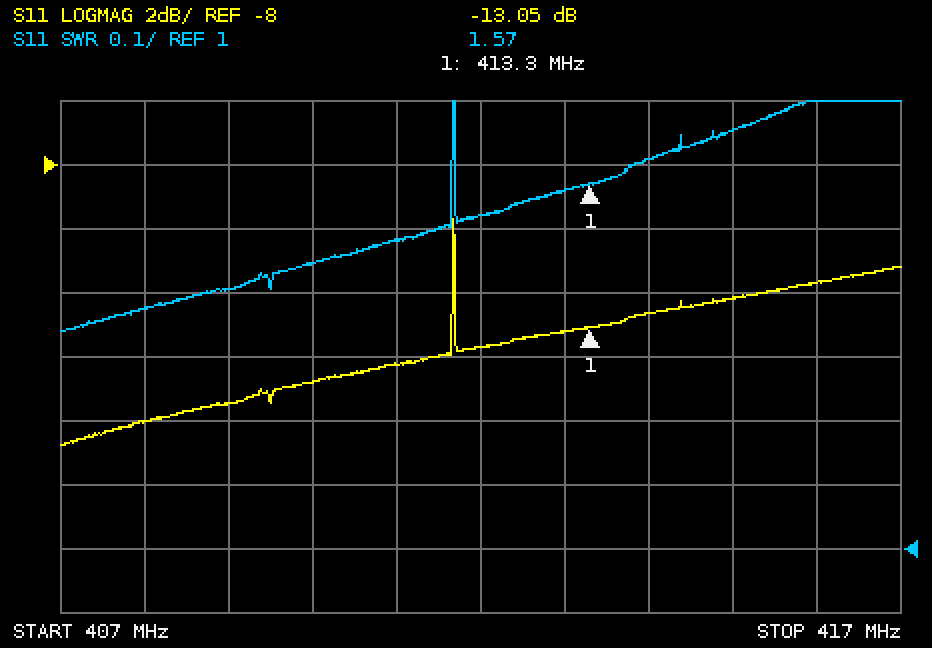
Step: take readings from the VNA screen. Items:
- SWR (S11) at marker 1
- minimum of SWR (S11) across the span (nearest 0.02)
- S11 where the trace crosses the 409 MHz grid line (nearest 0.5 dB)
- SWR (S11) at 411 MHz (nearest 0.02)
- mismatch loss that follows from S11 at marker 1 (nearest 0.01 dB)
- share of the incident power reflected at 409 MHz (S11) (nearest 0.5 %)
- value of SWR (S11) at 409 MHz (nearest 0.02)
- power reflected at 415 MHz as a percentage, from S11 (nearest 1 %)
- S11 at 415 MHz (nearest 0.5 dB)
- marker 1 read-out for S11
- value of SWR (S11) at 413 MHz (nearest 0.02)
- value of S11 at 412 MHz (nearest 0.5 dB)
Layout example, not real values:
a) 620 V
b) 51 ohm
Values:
a) 1.57
b) 1.34
c) -15.5 dB
d) 1.48
e) 0.22 dB
f) 3.0 %
g) 1.40
h) 6 %
i) -12.0 dB
j) -13.05 dB
k) 1.56
l) -13.5 dB
